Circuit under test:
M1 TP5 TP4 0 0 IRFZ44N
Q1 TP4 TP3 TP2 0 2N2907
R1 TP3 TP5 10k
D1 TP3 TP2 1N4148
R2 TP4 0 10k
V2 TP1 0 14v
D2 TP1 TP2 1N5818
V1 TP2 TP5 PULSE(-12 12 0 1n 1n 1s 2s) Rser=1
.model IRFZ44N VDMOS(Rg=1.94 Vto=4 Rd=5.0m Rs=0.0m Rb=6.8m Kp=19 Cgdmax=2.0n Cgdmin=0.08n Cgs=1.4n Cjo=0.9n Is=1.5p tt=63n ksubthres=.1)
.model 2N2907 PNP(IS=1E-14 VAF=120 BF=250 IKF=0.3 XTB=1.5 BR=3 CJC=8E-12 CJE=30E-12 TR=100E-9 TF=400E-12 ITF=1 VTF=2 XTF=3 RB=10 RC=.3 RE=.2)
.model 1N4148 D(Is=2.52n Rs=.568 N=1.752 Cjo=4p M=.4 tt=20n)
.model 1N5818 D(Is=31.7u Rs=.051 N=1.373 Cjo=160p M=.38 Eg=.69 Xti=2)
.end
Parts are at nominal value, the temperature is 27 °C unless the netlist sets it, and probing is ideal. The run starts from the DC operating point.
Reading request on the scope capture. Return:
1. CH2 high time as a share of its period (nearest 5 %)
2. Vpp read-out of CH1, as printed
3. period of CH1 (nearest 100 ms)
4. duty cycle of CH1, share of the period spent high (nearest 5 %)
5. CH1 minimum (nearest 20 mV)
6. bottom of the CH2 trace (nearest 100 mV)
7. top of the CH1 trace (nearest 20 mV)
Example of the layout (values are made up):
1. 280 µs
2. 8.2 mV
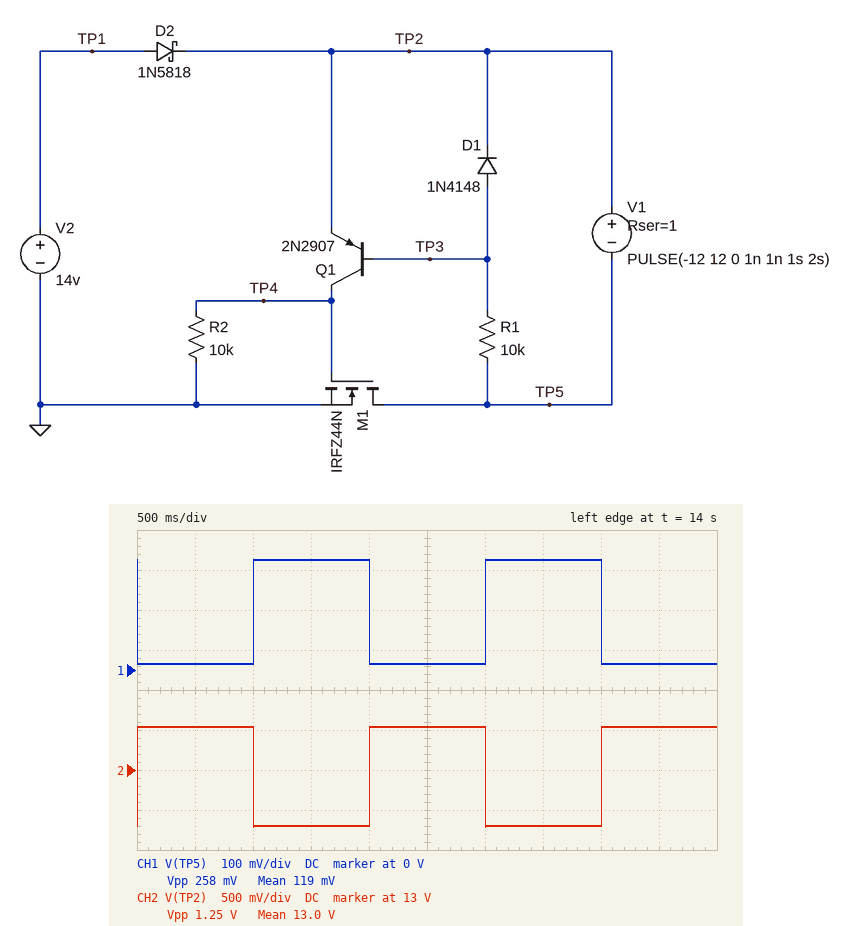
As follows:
1. 50 %
2. 258 mV
3. 2.0 s
4. 50 %
5. 20 mV
6. 12.3 V
7. 280 mV
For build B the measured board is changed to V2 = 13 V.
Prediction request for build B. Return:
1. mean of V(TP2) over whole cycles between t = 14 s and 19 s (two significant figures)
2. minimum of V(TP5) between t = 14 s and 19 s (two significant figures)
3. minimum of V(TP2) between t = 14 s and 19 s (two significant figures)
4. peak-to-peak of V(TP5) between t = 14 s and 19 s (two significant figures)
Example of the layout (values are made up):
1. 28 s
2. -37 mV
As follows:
1. 12 V
2. 6.8 mV
3. 11 V
4. 280 mV
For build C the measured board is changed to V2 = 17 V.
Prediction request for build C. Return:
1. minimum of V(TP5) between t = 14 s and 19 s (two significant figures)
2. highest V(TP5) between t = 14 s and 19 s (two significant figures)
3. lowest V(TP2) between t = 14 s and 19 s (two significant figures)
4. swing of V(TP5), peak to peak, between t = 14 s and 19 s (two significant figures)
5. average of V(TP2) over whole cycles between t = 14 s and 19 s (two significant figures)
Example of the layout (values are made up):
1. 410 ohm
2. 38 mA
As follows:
1. 40 mV
2. 260 mV
3. 15 V
4. 220 mV
5. 16 V
